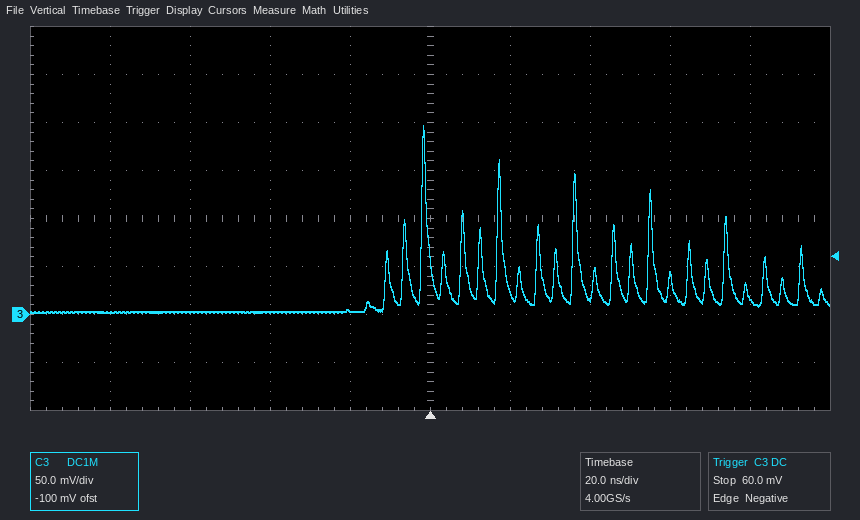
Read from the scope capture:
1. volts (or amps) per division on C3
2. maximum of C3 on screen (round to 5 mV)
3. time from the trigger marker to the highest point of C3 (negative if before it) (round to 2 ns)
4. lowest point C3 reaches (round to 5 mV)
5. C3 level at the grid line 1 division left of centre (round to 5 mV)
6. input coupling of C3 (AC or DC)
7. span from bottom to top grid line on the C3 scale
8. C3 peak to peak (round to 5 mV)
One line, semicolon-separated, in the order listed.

50 mV; 195 mV; -2 ns; 0 mV; 5 mV; DC; 400 mV; 195 mV
